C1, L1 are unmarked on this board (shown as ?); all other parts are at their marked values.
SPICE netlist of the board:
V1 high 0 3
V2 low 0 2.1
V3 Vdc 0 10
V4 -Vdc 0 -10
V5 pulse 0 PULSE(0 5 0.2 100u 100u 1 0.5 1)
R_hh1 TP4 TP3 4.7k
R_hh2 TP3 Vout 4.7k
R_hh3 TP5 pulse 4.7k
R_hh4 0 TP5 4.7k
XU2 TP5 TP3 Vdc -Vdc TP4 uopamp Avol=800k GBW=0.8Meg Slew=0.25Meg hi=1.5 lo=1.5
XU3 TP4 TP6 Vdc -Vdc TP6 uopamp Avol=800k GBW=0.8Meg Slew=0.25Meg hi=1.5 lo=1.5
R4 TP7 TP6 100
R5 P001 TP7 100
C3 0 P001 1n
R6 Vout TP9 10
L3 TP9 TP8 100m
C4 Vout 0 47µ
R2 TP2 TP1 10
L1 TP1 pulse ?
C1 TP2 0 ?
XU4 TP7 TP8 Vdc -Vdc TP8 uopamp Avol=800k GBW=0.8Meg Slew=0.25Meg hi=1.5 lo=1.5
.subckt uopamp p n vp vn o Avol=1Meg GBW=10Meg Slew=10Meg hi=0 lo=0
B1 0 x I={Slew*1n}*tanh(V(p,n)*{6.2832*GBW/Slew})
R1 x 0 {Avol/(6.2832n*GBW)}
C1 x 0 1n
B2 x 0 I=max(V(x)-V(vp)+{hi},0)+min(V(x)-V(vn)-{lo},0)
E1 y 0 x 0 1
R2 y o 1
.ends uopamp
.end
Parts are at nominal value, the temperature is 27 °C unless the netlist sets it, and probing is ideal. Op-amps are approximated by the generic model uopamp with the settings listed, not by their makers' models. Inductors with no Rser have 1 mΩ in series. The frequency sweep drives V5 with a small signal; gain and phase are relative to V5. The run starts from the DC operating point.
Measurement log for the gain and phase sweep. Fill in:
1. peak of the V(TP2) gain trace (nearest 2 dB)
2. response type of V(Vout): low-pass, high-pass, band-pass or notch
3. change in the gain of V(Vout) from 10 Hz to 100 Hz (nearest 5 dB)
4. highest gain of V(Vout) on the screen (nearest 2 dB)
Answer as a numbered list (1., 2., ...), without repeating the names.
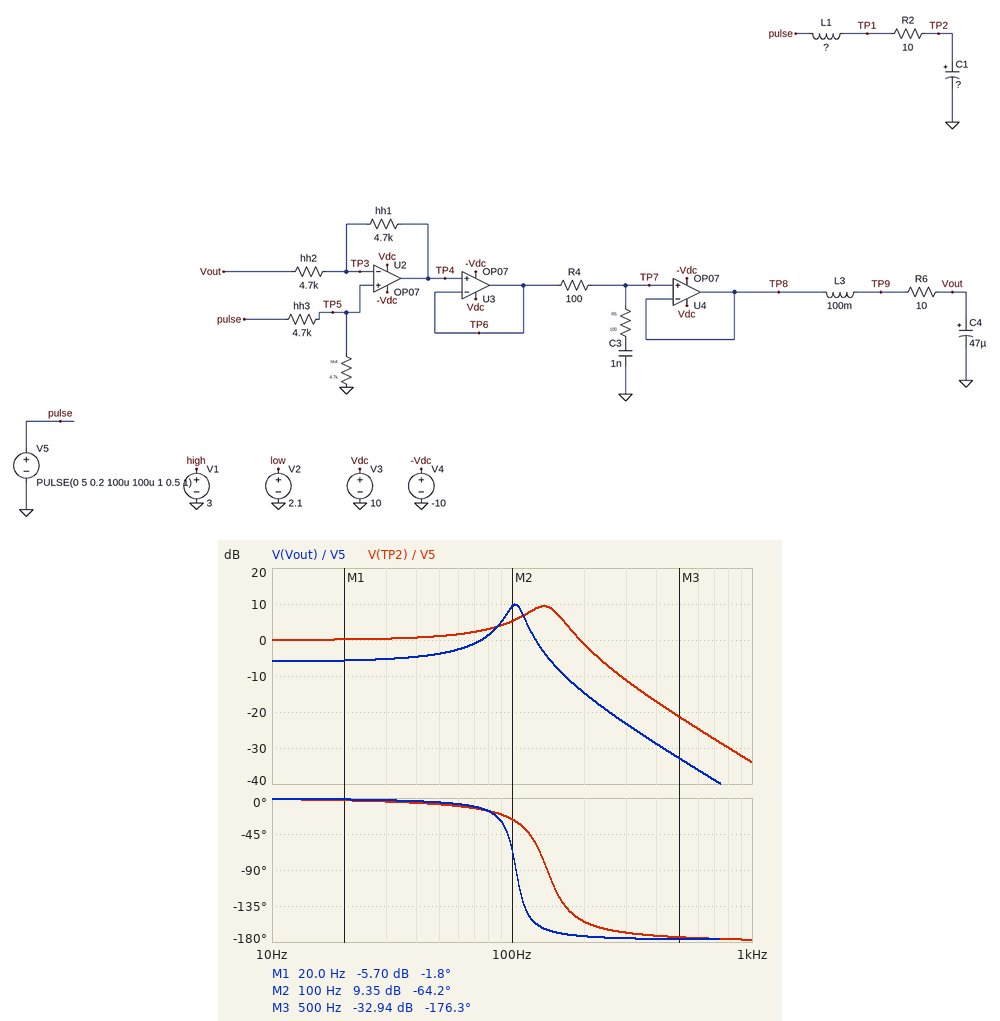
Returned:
1. 10 dB
2. low-pass
3. 15 dB
4. 10 dB
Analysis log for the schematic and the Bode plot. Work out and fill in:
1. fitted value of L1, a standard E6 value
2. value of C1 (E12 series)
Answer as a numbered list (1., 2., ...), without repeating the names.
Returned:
1. 33 mH
2. 39 µF
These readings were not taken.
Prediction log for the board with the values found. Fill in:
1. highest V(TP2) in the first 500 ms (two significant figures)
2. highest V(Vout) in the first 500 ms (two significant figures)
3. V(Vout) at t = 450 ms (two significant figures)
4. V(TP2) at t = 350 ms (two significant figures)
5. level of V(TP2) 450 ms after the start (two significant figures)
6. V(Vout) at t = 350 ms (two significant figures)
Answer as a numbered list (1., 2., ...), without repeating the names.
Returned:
1. 7.9 V
2. 4.4 V
3. 2.5 V
4. 5.0 V
5. 5.0 V
6. 2.5 V
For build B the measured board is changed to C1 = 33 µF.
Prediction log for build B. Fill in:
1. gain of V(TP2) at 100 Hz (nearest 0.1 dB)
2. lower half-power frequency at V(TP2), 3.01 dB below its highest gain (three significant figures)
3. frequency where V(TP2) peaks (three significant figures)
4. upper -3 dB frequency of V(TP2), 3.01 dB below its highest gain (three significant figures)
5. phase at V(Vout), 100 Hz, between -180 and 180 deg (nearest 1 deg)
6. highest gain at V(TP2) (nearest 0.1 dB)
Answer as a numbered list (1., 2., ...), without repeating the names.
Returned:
1. 4.3 dB
2. 122 Hz
3. 149 Hz
4. 171 Hz
5. -64 deg
6. 10.1 dB
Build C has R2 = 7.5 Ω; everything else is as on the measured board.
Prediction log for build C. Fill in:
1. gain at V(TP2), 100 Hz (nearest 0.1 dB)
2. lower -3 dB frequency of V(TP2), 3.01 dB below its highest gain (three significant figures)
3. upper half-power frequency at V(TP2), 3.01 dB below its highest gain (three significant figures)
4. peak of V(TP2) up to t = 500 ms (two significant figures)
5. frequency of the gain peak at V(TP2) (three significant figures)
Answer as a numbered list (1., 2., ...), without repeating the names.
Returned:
1. 5.6 dB
2. 118 Hz
3. 155 Hz
4. 8.3 V
5. 138 Hz
